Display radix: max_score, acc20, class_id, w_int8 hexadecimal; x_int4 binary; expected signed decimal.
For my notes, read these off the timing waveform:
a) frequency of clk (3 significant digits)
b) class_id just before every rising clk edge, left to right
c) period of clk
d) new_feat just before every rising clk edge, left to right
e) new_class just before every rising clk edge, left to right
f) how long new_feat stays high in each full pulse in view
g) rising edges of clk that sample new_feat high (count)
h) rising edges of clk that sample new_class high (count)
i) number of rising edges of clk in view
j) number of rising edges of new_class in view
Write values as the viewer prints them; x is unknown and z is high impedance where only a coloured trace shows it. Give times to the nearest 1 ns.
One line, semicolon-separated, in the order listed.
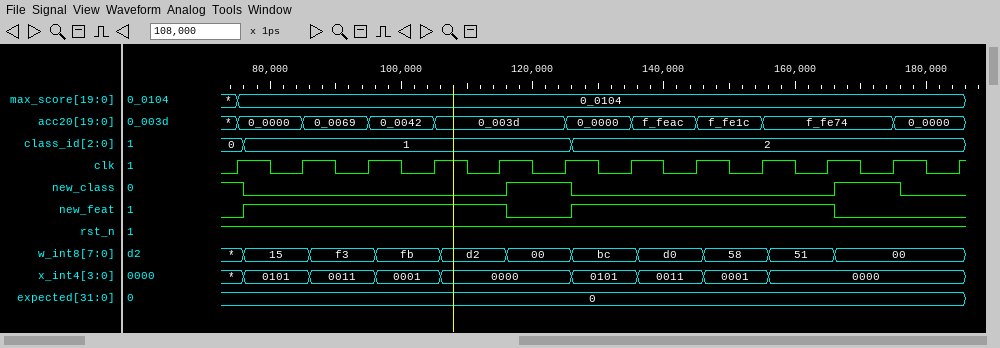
100 MHz; 0, 1, 1, 1, 1, 1, 2, 2, 2, 2, 2, 2; 10 ns; 0 1 1 1 1 0 1 1 1 1 0 0; 1 0 0 0 0 1 0 0 0 0 1 0; 40 ns, 40 ns; 8; 3; 12; 2
